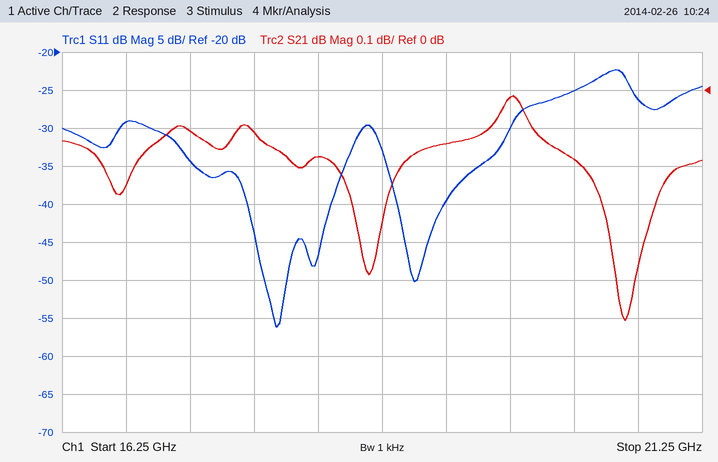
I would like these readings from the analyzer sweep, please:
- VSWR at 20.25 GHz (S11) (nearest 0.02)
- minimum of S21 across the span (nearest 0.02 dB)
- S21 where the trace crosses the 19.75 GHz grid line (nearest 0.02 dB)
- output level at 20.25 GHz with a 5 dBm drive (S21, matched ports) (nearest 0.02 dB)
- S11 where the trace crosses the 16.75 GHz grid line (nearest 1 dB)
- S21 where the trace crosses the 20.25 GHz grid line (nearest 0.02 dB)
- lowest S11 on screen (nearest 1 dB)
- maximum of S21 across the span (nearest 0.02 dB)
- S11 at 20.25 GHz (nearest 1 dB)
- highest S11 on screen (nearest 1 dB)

1.12
-0.60 dB
-0.02 dB
4.82 dBm
-29 dB
-0.18 dB
-56 dB
-0.02 dB
-25 dB
-22 dB
